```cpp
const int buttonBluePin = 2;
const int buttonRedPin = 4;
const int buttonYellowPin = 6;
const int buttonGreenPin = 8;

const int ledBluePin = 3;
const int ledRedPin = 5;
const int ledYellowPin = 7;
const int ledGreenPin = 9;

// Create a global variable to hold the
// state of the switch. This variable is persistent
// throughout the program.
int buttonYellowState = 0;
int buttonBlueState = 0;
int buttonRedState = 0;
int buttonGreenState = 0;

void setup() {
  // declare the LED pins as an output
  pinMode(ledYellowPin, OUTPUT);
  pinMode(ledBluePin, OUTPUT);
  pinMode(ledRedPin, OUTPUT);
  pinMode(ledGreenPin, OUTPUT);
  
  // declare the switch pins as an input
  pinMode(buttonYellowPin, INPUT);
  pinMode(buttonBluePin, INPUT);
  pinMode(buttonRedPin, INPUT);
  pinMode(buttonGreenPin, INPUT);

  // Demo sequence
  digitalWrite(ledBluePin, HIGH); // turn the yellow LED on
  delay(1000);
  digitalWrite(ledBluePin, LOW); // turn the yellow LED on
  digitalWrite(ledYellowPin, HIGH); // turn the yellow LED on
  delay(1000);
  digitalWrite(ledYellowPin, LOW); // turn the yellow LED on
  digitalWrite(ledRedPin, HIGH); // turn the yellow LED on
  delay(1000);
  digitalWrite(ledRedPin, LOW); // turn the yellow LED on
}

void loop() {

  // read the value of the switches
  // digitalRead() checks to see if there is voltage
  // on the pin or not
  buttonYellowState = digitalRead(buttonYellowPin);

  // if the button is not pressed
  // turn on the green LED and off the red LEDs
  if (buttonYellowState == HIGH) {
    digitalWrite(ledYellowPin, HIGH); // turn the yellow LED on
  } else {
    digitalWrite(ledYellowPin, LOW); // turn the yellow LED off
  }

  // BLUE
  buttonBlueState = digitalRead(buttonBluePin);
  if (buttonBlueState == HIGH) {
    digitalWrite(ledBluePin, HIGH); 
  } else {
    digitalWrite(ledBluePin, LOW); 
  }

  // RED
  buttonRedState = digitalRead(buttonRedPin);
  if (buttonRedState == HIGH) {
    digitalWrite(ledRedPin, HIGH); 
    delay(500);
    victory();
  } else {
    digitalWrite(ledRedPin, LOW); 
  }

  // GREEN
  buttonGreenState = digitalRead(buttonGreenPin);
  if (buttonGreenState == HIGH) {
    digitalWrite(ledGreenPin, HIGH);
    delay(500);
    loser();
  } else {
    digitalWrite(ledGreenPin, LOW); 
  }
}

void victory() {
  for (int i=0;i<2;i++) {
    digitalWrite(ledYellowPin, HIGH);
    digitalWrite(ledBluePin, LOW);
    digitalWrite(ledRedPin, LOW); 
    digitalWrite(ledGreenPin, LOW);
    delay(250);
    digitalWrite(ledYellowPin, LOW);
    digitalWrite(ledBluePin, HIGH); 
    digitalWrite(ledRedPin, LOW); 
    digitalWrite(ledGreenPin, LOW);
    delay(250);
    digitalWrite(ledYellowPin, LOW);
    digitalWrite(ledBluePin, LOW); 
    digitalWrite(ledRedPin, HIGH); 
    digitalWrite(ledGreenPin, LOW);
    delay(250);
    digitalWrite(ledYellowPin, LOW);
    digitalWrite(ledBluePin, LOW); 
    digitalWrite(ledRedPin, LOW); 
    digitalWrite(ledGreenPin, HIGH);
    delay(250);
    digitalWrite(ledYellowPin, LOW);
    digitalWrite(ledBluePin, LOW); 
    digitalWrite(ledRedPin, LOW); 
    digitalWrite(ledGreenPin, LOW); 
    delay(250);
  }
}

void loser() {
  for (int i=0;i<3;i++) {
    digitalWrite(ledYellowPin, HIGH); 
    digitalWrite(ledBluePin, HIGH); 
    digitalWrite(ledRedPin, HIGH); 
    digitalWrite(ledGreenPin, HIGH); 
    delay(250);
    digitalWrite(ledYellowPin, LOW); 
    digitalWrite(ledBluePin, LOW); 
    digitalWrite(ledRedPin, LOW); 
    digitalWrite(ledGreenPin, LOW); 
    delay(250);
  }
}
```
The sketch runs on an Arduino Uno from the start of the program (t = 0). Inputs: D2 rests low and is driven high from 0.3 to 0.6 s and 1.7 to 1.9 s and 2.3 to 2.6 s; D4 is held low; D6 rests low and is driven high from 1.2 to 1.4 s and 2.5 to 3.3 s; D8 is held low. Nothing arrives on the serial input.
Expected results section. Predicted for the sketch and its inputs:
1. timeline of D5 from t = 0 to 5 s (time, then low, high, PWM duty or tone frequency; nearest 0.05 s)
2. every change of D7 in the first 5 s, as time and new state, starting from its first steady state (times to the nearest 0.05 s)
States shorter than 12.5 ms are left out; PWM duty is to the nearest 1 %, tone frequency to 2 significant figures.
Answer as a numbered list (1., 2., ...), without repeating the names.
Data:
1. 0 s low; 2 s high; 3 s low
2. 0 s low; 1 s high; 2 s low; 3 s high; 3.3 s low
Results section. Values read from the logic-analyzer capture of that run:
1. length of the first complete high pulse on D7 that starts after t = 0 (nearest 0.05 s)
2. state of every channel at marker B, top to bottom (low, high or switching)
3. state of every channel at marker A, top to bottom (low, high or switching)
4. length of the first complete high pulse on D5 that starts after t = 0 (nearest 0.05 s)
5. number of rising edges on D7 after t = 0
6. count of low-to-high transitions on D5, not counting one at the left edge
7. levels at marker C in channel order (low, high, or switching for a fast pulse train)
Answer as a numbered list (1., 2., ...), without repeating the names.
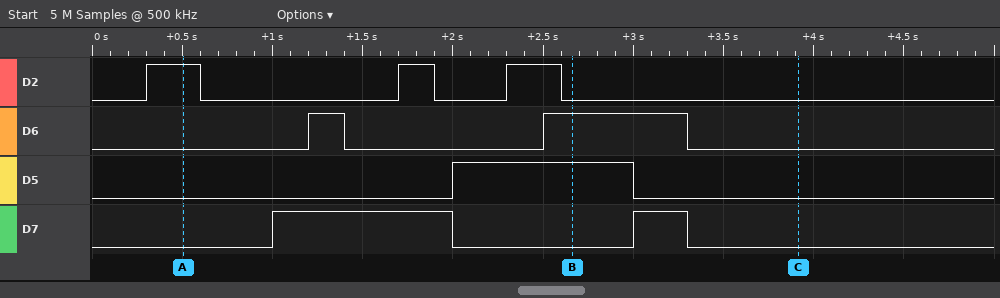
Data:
1. 1.00 s
2. D2 low, D6 high, D5 high, D7 low
3. D2 high, D6 low, D5 low, D7 low
4. 1.00 s
5. 2
6. 1
7. D2 low, D6 low, D5 low, D7 low
